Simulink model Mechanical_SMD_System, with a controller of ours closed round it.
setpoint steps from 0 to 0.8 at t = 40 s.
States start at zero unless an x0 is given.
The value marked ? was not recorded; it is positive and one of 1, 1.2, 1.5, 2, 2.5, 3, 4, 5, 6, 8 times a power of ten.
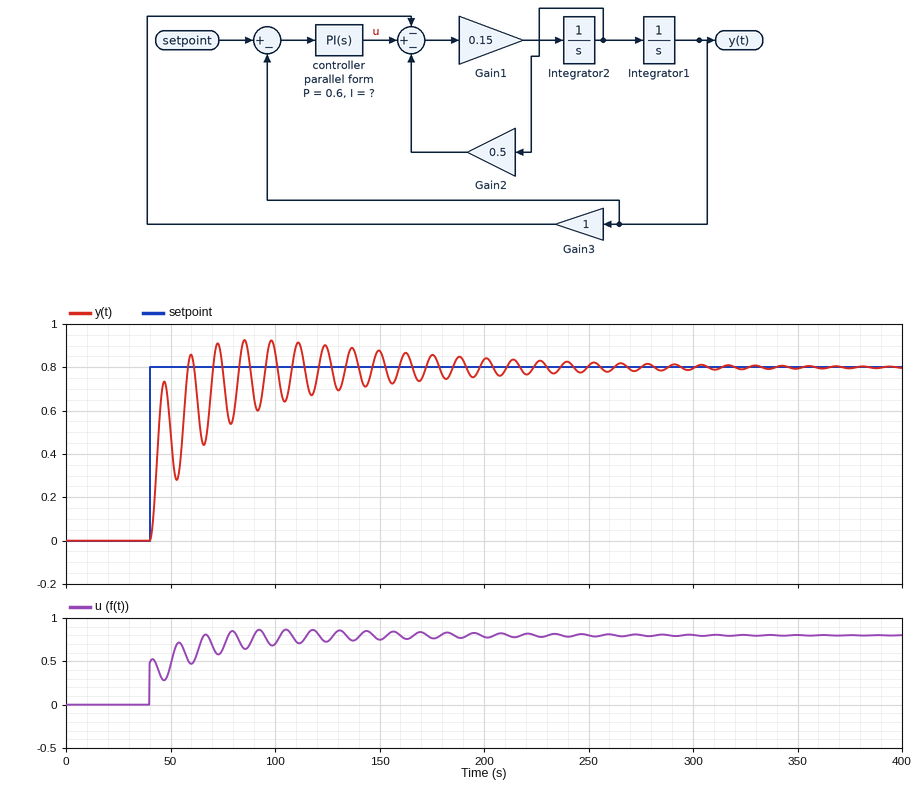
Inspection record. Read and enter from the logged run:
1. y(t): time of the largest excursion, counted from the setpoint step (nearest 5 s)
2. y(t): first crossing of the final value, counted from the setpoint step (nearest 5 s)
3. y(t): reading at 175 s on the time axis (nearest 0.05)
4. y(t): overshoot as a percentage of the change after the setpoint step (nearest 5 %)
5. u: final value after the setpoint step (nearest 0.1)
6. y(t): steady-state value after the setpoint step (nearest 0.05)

45 s
20 s
0.85
15 %
0.8
0.80
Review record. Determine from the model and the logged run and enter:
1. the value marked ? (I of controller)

0.08
